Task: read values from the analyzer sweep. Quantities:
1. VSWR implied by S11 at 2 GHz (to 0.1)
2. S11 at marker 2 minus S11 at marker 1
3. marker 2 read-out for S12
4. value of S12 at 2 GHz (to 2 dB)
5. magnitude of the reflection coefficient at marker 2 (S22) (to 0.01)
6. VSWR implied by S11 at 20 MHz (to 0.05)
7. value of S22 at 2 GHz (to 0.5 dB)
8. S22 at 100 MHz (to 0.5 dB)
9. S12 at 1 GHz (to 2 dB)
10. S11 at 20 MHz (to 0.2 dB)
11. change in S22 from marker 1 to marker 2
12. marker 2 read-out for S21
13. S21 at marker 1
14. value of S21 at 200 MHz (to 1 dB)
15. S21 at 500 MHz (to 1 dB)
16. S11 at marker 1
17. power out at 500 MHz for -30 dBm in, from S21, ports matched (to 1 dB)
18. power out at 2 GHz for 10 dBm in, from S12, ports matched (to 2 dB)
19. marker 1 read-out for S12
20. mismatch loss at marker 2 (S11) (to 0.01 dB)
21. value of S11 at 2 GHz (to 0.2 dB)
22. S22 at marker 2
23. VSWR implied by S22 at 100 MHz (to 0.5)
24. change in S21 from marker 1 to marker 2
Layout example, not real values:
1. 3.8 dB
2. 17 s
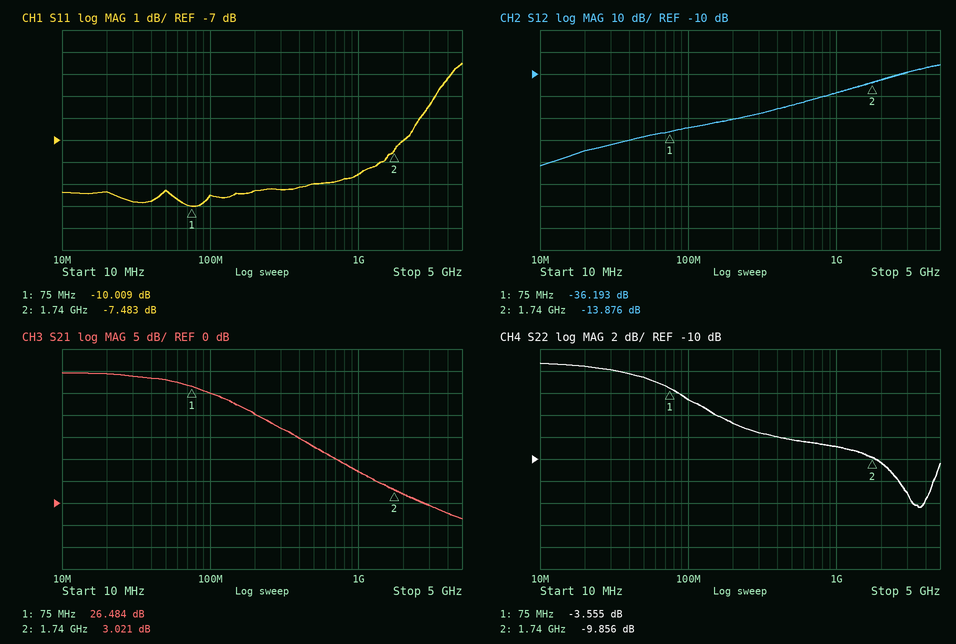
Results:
1. 2.6
2. 2.526 dB
3. -13.876 dB
4. -12 dB
5. 0.32
6. 2.05
7. -10.5 dB
8. -4.5 dB
9. -18 dB
10. -9.4 dB
11. -6.301 dB
12. 3.021 dB
13. 26.484 dB
14. 20 dB
15. 13 dB
16. -10.009 dB
17. -17 dBm
18. -2 dBm
19. -36.193 dB
20. 0.85 dB
21. -7.0 dB
22. -9.856 dB
23. 4.0
24. -23.463 dB
